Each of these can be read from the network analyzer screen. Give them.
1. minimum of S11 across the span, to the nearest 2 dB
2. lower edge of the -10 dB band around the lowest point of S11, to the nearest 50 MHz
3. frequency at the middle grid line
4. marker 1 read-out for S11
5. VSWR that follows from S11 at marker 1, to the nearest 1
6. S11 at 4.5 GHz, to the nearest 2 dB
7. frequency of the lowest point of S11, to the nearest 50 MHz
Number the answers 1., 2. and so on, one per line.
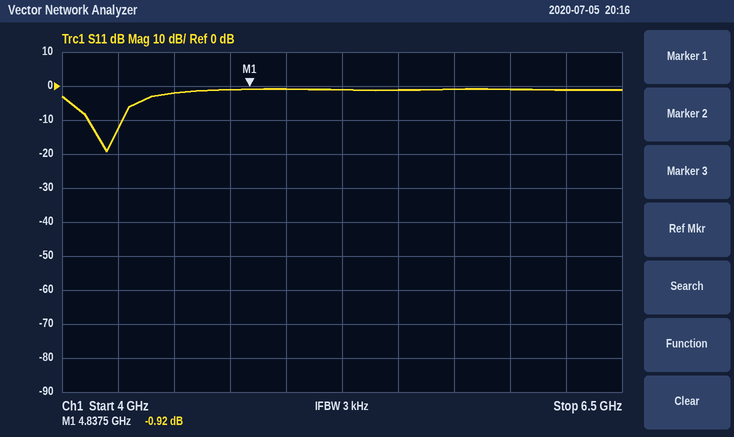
1. -20 dB
2. 4.10 GHz
3. 5.25 GHz
4. -0.92 dB
5. 19
6. -2 dB
7. 4.20 GHz
